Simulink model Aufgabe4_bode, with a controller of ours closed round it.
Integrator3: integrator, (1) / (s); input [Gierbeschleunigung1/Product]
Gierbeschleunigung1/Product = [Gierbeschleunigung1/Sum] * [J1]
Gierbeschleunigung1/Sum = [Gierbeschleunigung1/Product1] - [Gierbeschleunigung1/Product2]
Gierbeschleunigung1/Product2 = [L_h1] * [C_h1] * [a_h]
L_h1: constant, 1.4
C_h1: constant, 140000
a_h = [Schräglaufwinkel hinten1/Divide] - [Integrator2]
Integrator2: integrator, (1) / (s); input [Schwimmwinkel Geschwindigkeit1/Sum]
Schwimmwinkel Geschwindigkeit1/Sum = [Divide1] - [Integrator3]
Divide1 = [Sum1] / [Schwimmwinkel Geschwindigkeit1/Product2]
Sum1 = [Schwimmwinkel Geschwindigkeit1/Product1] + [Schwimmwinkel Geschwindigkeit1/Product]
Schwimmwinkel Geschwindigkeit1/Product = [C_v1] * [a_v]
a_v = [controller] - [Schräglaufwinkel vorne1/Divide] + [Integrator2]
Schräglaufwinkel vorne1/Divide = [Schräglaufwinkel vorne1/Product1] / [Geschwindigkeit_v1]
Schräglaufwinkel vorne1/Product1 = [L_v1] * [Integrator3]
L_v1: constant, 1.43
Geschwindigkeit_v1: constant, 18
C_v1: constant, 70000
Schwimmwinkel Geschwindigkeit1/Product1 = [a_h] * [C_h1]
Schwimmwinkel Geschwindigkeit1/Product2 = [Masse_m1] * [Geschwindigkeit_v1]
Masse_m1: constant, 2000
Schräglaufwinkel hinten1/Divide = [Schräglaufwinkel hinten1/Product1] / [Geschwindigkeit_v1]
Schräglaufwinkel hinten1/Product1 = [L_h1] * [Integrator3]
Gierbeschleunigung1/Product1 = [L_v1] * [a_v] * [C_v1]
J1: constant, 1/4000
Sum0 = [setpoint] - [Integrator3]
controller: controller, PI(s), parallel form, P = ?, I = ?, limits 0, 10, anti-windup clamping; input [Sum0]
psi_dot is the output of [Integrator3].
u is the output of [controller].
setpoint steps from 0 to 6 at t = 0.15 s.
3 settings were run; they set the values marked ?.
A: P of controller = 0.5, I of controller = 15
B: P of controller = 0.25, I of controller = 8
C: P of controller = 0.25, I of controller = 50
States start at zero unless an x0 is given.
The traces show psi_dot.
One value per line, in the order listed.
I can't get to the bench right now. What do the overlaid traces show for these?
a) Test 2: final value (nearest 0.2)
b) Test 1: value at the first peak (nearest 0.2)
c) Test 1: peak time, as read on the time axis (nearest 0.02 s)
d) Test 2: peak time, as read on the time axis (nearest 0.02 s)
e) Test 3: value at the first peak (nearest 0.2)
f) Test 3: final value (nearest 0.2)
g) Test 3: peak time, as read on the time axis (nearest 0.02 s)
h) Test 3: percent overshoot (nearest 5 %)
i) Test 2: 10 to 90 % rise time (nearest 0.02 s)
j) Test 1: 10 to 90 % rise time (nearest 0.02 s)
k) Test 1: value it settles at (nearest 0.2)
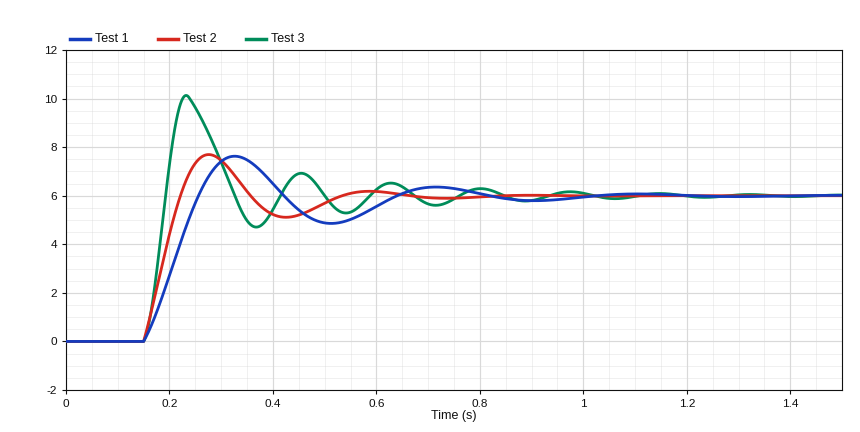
6.0
7.6
0.32 s
0.28 s
10.2
6.0
0.24 s
70 %
0.06 s
0.08 s
6.0
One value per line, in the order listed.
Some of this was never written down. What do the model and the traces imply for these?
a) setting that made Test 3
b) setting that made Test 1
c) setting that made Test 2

C
B
A
